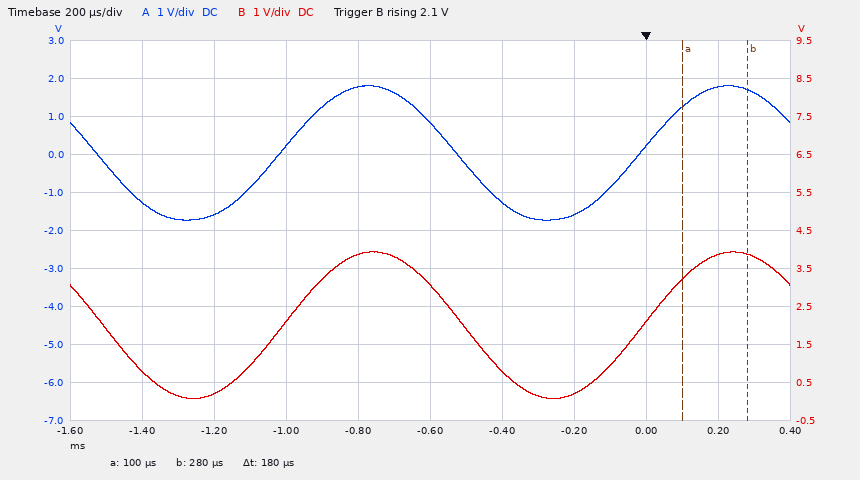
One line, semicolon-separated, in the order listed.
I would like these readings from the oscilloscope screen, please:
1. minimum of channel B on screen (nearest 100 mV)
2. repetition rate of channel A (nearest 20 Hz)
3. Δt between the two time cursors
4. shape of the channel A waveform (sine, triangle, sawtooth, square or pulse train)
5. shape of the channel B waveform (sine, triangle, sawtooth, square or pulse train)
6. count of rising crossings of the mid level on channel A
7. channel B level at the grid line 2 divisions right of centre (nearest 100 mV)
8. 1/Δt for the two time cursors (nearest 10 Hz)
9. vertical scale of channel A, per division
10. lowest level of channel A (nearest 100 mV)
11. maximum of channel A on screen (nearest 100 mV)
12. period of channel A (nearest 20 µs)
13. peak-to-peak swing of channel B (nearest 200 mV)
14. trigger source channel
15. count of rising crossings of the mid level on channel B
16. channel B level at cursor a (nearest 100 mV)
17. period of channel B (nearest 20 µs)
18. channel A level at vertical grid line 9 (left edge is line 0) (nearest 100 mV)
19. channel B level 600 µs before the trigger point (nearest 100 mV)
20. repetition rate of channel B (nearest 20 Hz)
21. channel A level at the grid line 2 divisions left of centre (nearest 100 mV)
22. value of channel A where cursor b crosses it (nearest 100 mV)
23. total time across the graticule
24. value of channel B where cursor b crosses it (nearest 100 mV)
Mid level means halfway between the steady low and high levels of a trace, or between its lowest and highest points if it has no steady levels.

100 mV; 1.00 kHz; 180 µs; sine; sine; 2; 200 mV; 5.56 kHz; 1 V; -1.7 V; 1.8 V; 1.00 ms; 3.8 V; channel B; 2; 3.2 V; 1.00 ms; 1.8 V; 3.1 V; 1.00 kHz; 200 mV; 1.7 V; 2 ms; 3.9 V
